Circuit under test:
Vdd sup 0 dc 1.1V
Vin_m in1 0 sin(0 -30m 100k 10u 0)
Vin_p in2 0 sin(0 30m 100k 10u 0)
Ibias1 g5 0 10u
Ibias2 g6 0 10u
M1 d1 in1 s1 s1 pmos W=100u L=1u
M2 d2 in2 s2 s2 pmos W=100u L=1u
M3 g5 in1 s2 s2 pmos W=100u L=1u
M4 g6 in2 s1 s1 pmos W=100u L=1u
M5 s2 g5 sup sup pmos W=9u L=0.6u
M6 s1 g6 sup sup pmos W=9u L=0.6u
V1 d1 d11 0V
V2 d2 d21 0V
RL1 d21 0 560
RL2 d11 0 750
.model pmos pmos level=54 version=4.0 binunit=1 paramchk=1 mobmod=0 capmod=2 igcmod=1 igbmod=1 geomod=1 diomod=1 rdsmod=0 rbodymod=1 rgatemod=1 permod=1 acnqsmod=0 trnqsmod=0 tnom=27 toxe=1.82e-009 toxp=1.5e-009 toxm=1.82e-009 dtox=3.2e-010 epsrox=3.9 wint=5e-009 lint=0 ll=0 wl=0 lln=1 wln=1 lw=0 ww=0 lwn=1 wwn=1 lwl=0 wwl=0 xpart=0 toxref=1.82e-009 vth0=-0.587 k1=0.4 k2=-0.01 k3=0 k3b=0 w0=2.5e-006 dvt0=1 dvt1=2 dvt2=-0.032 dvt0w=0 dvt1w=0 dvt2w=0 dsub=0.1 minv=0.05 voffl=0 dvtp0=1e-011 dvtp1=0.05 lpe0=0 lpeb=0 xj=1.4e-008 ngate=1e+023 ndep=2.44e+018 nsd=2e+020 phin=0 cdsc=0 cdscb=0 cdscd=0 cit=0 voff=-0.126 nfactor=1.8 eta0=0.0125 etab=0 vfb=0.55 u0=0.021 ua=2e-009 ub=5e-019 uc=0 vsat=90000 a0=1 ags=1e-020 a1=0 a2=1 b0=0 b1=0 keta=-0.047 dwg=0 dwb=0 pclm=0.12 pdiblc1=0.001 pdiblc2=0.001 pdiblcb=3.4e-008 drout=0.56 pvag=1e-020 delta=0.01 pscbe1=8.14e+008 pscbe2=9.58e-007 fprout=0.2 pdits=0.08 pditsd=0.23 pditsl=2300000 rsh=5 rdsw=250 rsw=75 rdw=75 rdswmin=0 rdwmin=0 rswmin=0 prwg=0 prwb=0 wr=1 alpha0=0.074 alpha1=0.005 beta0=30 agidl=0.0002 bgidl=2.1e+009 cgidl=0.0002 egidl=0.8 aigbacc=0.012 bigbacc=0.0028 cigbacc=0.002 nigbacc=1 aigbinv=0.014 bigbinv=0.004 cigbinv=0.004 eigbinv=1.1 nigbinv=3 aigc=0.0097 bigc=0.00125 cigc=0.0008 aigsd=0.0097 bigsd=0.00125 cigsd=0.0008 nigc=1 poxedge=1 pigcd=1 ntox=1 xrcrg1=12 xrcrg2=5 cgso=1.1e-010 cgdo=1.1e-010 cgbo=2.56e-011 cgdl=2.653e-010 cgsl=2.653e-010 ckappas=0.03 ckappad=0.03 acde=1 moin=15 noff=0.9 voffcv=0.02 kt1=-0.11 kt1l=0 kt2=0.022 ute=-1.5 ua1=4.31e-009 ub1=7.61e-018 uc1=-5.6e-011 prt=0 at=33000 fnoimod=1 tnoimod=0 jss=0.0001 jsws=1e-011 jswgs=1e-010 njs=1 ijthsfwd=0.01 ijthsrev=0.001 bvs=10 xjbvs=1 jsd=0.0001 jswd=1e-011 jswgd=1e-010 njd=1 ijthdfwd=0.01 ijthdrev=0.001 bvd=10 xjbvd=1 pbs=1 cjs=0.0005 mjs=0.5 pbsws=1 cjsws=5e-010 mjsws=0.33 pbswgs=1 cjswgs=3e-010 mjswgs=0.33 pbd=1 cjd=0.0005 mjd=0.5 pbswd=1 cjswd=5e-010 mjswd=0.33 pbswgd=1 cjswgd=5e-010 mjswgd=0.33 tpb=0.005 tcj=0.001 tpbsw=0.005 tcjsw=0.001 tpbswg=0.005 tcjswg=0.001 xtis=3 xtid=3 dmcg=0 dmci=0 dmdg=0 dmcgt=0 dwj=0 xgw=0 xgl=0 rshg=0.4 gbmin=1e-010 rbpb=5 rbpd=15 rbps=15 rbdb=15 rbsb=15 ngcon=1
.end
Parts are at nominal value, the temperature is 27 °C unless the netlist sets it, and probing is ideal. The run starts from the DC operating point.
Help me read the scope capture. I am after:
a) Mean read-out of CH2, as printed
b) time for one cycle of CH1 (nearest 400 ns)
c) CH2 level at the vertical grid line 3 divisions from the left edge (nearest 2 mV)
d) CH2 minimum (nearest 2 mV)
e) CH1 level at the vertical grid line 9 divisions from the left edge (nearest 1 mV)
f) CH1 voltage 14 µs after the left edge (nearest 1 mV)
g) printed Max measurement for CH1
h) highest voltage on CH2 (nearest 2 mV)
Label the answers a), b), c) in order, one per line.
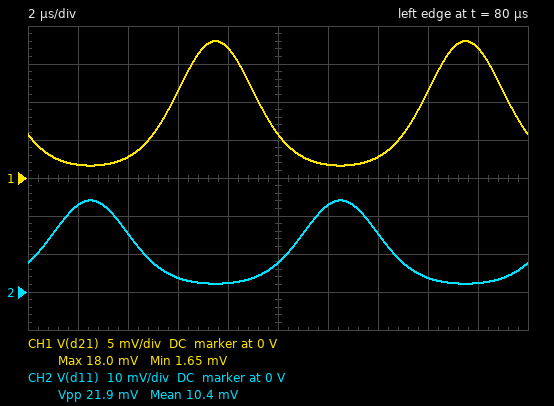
a) 10.4 mV
b) 10.0 µs
c) 4 mV
d) 2 mV
e) 17 mV
f) 3 mV
g) 18.0 mV
h) 24 mV
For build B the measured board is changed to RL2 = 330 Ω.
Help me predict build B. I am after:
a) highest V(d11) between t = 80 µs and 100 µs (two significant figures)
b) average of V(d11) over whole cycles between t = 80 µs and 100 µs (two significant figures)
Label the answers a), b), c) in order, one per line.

a) 11 mV
b) 4.6 mV
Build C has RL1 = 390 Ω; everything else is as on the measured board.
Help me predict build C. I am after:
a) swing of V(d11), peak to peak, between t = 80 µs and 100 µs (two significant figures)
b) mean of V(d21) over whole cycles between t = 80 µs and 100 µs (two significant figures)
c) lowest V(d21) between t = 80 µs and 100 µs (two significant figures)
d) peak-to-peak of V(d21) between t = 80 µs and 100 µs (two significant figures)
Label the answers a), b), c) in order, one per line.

a) 22 mV
b) 5.4 mV
c) 1.1 mV
d) 11 mV
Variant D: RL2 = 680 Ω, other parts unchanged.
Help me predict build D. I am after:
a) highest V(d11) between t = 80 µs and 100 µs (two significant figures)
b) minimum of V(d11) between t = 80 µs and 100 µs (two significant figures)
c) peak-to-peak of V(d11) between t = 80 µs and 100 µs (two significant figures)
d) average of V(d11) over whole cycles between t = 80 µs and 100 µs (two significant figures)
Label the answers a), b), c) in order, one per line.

a) 22 mV
b) 2.0 mV
c) 20 mV
d) 9.4 mV
